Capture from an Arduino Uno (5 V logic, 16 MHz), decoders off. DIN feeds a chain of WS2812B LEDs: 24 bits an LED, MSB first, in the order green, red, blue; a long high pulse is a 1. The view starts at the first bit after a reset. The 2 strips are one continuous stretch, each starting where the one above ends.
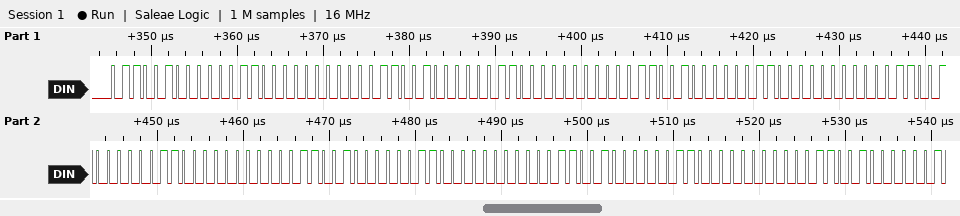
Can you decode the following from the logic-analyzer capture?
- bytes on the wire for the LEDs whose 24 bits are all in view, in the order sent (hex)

64 0C 00 64 0C 00 64 0C 00 64 0C 00 64 0C 00 64 0C 00
